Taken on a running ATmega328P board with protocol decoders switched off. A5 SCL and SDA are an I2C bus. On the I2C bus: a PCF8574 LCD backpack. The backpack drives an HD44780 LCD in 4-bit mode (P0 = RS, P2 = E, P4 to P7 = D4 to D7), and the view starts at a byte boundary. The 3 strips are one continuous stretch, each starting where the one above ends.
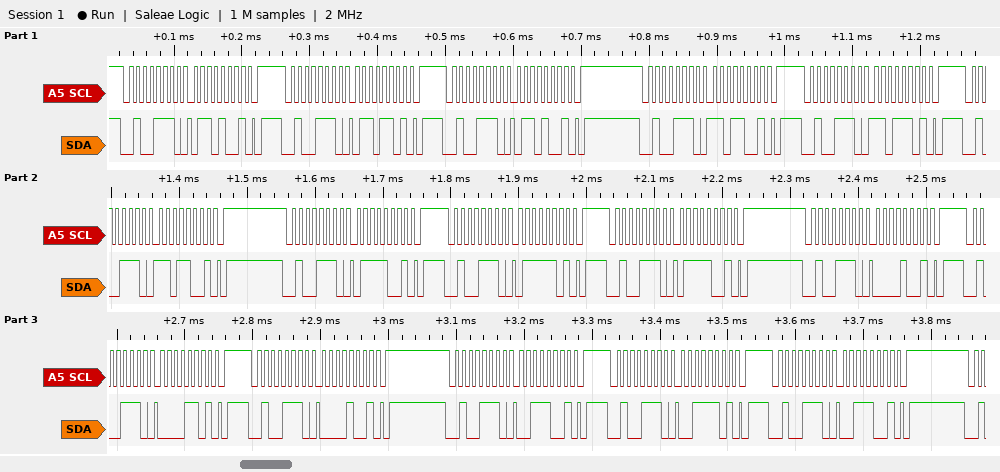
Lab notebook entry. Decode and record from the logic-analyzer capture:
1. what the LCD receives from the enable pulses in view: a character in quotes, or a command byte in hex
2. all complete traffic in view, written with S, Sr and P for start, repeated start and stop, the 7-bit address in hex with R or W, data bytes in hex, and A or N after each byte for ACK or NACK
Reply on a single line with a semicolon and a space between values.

'm' 'p'; S 27W A 69 A P S 27W A 6D A P S 27W A 69 A P S 27W A D9 A P S 27W A DD A P S 27W A D9 A P S 27W A 79 A P S 27W A 7D A P S 27W A 79 A P S 27W A 09 A P S 27W A 0D A P S 27W A 09 A P S 27W A 39 A P S 27W A 3D A P S 27W A 39 A P
